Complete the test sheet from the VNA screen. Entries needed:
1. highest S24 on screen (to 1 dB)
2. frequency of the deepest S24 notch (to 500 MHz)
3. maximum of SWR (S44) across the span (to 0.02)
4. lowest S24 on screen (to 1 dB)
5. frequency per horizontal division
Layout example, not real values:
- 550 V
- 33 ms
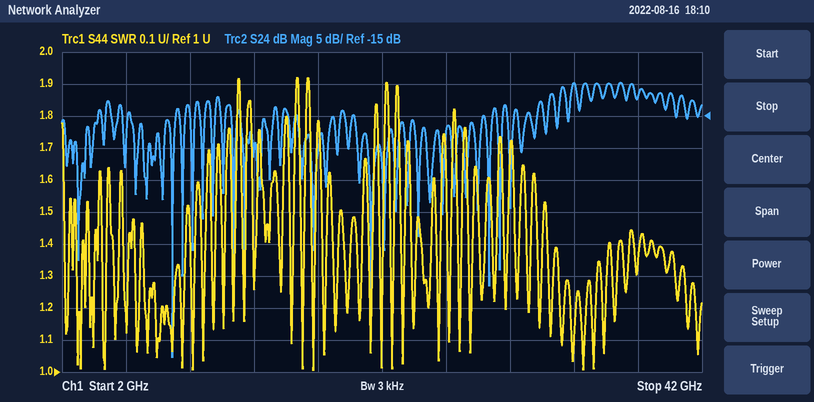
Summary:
- -10 dB
- 9.0 GHz
- 1.92
- -53 dB
- 4 GHz
